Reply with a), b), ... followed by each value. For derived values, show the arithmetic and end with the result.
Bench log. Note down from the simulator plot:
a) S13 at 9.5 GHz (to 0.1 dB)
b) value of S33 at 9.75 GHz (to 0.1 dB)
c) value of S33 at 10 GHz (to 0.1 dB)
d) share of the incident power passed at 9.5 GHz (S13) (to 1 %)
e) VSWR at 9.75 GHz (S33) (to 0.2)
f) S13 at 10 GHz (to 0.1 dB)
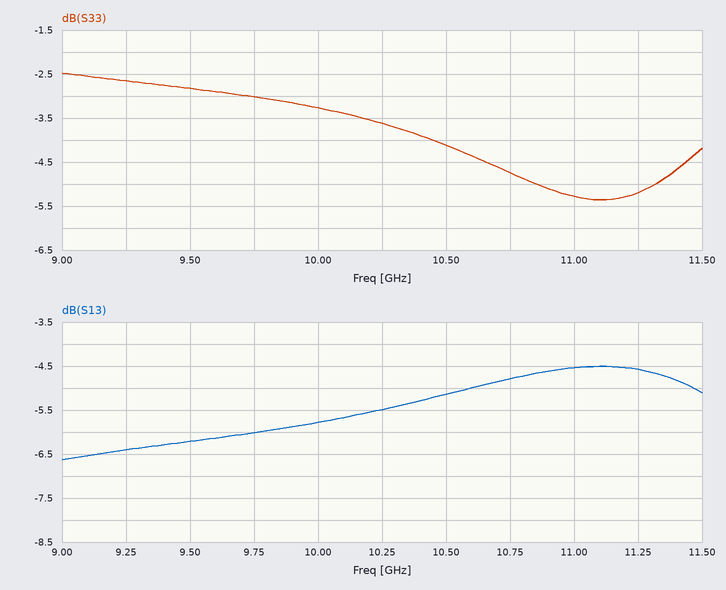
a) -6.2 dB
b) -3.0 dB
c) -3.3 dB
d) 10^(-6.2/10) ≈ 24 %
e) |Γ| = 10^(-3/20) = 0.7079; VSWR = (1 + 0.7079)/(1 − 0.7079) ≈ 5.8
f) -5.8 dB
